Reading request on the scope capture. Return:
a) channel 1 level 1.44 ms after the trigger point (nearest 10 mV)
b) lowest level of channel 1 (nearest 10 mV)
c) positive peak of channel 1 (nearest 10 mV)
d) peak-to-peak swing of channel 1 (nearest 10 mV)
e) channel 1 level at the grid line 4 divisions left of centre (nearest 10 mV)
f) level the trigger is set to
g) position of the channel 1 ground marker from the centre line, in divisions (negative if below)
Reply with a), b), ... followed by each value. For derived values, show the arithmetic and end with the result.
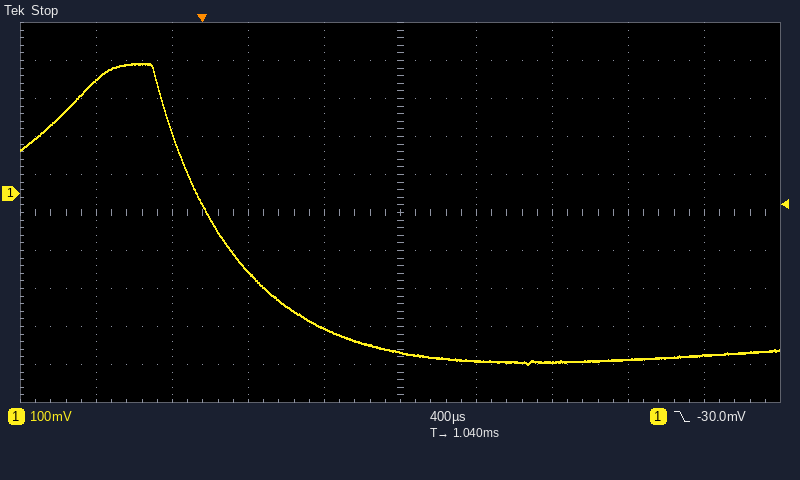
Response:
a) -440 mV
b) -450 mV
c) 340 mV
d) 340 mV − (-450 mV) = 790 mV
e) 300 mV
f) -30.0 mV
g) +0.5 div
